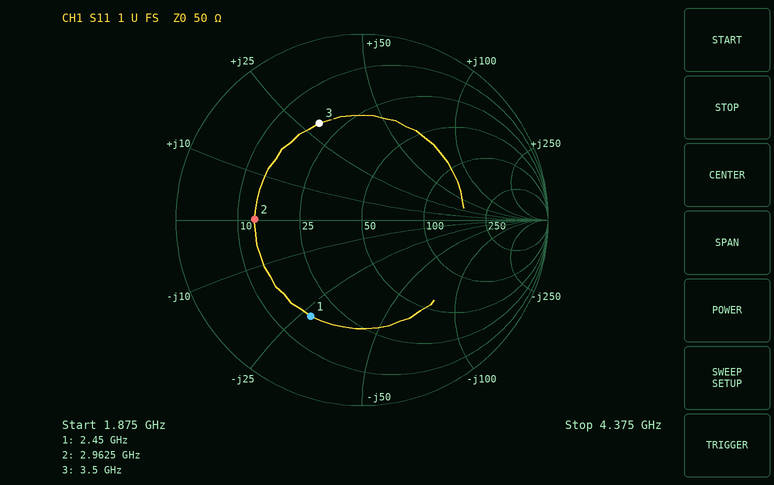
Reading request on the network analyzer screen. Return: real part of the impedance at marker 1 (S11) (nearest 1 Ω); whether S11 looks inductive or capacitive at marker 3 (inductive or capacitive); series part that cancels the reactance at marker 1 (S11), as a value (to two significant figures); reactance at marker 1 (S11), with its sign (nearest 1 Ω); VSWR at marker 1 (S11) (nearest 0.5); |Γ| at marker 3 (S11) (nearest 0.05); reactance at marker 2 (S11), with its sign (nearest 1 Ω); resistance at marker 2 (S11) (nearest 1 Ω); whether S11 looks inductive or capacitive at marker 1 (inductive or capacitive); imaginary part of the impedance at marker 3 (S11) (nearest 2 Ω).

17 Ω
inductive
1.8 nH
-27 Ω
4.0
0.55
0 Ω
13 Ω
capacitive
+30 Ω
